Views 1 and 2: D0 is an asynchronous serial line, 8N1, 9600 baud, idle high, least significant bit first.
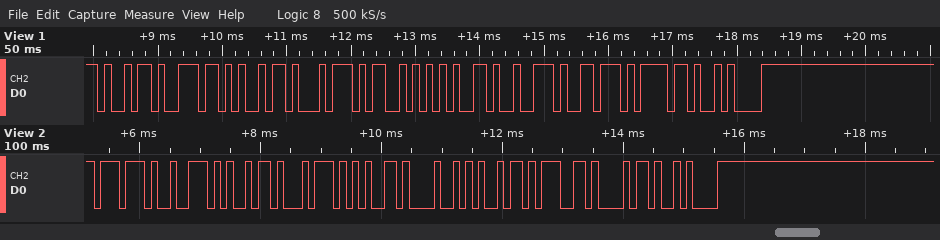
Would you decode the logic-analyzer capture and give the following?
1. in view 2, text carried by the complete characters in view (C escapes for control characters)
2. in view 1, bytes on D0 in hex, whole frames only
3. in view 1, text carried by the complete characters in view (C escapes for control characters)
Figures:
"writeHigh\n"
69 6E 69 74 53 65 72 76 6F 0A
"initServo\n"
